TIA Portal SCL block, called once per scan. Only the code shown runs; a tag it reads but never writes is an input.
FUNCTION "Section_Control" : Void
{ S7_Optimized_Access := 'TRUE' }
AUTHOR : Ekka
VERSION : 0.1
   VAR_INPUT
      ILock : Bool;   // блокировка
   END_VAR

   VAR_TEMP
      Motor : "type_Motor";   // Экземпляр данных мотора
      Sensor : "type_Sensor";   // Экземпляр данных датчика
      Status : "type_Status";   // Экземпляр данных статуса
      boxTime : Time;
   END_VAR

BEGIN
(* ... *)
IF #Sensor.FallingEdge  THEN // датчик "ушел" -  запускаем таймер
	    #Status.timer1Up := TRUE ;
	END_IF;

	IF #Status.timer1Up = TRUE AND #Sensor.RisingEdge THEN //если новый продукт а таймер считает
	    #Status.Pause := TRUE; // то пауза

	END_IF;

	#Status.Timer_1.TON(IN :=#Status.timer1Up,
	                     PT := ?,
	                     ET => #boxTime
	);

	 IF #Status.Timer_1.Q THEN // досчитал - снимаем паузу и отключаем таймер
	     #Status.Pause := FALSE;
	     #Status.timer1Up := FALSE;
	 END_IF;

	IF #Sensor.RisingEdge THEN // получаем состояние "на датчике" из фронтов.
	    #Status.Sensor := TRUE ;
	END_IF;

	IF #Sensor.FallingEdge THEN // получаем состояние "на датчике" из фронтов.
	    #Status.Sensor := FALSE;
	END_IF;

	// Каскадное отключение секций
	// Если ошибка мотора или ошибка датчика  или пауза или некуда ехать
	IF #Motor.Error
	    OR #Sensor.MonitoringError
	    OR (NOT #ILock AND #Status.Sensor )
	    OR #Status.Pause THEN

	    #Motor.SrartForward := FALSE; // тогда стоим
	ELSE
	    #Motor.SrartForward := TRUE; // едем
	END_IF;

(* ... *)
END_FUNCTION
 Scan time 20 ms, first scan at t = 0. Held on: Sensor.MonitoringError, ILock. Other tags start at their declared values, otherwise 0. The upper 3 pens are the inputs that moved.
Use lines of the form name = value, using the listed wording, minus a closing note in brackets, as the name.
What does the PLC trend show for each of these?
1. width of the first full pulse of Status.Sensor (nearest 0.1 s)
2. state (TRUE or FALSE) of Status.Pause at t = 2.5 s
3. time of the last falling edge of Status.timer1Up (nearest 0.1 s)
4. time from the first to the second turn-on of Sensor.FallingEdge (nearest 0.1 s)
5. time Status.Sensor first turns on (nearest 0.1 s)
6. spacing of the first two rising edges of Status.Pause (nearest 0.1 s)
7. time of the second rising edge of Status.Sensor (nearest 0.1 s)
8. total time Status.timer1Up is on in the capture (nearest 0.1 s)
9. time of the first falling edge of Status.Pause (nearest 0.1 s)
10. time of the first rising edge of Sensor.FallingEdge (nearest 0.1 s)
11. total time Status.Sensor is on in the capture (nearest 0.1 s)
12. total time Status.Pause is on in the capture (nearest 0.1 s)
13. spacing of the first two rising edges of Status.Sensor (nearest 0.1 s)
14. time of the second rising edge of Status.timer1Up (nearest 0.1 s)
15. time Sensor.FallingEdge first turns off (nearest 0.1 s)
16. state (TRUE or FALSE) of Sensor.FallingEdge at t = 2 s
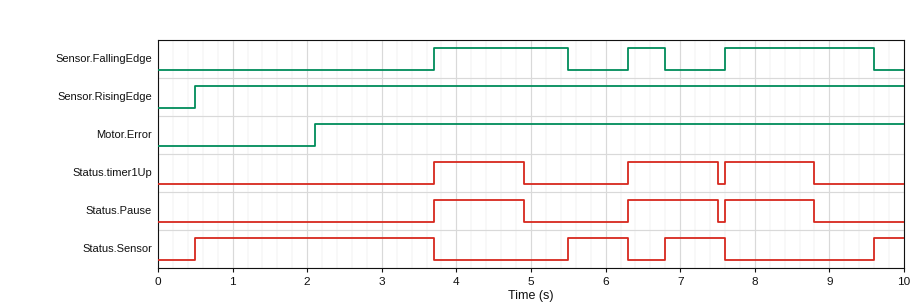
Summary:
width of the first full pulse of Status.Sensor = 3.2 s
state (TRUE or FALSE) of Status.Pause at t = 2.5 s = FALSE
time of the last falling edge of Status.timer1Up = 8.8 s
time from the first to the second turn-on of Sensor.FallingEdge = 2.6 s
time Status.Sensor first turns on = 0.5 s
spacing of the first two rising edges of Status.Pause = 2.6 s
time of the second rising edge of Status.Sensor = 5.5 s
total time Status.timer1Up is on in the capture = 3.6 s
time of the first falling edge of Status.Pause = 4.9 s
time of the first rising edge of Sensor.FallingEdge = 3.7 s
total time Status.Sensor is on in the capture = 5.2 s
total time Status.Pause is on in the capture = 3.6 s
spacing of the first two rising edges of Status.Sensor = 5.0 s
time of the second rising edge of Status.timer1Up = 6.3 s
time Sensor.FallingEdge first turns off = 5.5 s
state (TRUE or FALSE) of Sensor.FallingEdge at t = 2 s = FALSE
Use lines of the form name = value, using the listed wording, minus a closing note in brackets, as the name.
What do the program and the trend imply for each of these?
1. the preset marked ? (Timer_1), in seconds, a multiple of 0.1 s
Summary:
the preset marked ? (Timer_1), in seconds, a multiple of 0.1 s = 1.2 s
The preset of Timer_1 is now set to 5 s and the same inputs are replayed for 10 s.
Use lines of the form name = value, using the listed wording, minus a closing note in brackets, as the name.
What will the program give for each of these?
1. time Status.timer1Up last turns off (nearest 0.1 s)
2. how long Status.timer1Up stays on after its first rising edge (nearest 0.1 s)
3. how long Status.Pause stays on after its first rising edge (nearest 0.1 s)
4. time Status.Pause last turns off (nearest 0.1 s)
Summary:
time Status.timer1Up last turns off = 8.7 s
how long Status.timer1Up stays on after its first rising edge = 5.0 s
how long Status.Pause stays on after its first rising edge = 5.0 s
time Status.Pause last turns off = 8.7 s
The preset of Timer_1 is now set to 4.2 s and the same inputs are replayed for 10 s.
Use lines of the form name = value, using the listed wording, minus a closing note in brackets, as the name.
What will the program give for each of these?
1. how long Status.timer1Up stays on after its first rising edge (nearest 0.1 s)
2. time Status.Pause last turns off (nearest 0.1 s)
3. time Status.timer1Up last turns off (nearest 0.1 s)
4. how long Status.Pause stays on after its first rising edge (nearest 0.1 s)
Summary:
how long Status.timer1Up stays on after its first rising edge = 4.2 s
time Status.Pause last turns off = 7.9 s
time Status.timer1Up last turns off = 7.9 s
how long Status.Pause stays on after its first rising edge = 4.2 s
